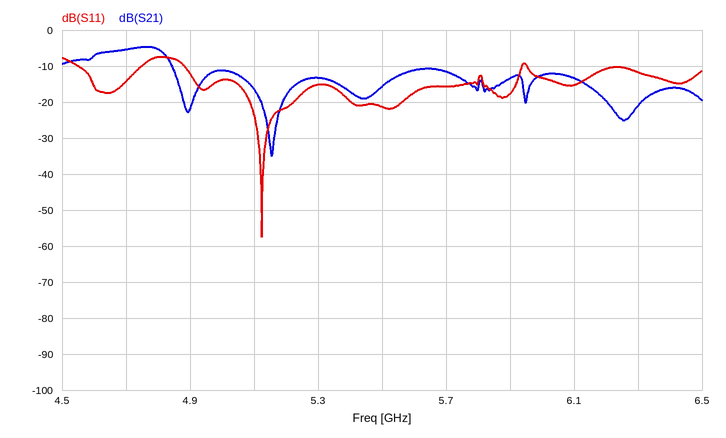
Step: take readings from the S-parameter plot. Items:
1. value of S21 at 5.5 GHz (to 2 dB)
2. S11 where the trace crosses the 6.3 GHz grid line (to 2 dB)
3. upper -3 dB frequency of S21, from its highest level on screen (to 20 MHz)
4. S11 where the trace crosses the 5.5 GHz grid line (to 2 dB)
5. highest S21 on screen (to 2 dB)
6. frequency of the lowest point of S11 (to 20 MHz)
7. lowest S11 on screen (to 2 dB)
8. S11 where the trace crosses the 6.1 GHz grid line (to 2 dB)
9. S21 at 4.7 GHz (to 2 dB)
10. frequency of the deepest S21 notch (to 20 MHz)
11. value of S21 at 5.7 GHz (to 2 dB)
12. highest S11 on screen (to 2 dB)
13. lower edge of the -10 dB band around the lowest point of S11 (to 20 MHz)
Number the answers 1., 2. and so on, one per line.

1. -16 dB
2. -12 dB
3. 4.82 GHz
4. -22 dB
5. -4 dB
6. 5.12 GHz
7. -58 dB
8. -16 dB
9. -6 dB
10. 5.16 GHz
11. -12 dB
12. -8 dB
13. 4.88 GHz
